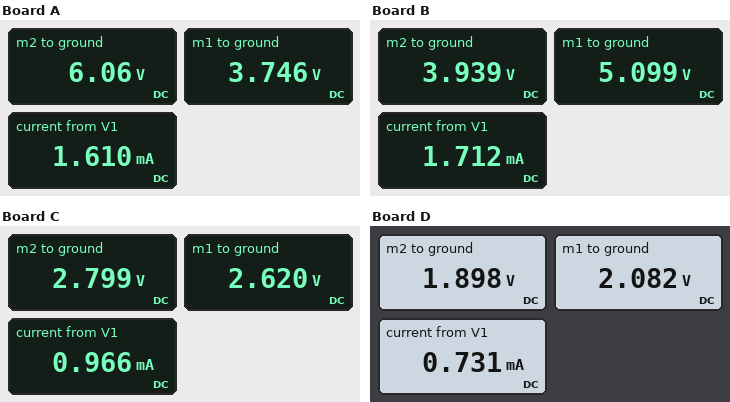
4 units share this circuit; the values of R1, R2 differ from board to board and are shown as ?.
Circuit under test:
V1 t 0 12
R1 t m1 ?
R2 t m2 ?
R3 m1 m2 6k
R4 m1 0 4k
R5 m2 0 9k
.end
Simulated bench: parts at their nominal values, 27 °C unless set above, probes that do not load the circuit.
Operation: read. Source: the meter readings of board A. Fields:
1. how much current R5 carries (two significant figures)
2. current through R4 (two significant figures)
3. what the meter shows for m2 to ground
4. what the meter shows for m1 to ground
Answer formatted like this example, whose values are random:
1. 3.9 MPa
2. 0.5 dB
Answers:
1. 670 µA
2. 940 µA
3. 6.06 V
4. 3.746 V
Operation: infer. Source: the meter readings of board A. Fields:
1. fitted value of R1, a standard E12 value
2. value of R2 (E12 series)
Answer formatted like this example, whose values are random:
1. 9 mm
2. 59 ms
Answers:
1. 15 kΩ
2. 5.6 kΩ
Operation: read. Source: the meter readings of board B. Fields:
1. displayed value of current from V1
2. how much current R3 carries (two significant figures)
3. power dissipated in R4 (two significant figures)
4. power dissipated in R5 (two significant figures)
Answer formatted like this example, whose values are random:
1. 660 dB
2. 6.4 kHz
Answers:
1. 1.712 mA
2. 190 µA
3. 6.5 mW
4. 1.7 mW
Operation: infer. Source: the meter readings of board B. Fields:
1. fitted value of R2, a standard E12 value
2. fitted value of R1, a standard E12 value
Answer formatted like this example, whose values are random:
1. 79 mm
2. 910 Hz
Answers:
1. 33 kΩ
2. 4.7 kΩ
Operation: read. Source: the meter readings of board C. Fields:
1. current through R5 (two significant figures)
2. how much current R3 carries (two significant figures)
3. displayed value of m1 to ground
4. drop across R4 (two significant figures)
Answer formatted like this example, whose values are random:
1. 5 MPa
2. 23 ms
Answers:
1. 310 µA
2. 30 µA
3. 2.620 V
4. 2.6 V
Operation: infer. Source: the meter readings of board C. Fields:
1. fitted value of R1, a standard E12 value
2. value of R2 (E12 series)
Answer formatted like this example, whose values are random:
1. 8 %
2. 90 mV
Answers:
1. 15 kΩ
2. 27 kΩ
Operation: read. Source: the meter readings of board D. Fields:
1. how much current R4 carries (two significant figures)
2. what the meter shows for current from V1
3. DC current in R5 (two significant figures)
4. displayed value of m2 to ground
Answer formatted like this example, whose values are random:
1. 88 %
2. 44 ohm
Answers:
1. 520 µA
2. 0.731 mA
3. 210 µA
4. 1.898 V
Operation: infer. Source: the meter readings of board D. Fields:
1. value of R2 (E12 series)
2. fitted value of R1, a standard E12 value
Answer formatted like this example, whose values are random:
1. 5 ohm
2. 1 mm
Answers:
1. 56 kΩ
2. 18 kΩ
